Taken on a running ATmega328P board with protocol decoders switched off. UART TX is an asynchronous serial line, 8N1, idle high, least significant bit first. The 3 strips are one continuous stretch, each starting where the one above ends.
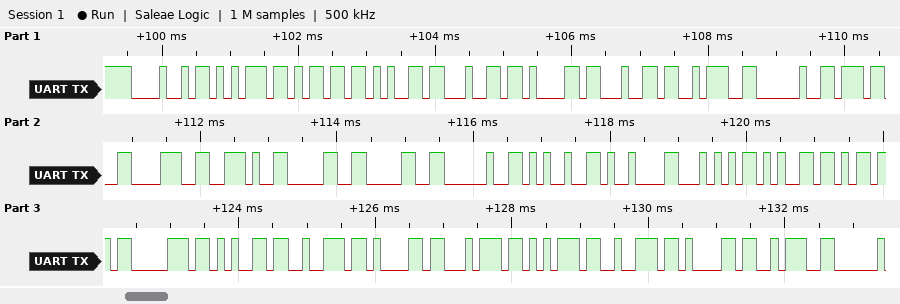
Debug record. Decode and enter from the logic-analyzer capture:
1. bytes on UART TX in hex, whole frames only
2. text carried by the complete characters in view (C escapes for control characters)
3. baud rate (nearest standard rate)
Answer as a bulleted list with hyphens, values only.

- 48 75 6D 65 64 61 64 3A 20 37 38 2E 30 30 20 25 09 54 65 6D 70 65 72 61 74 75 72 61 3A
- "Humedad: 78.00 %\tTemperatura:"
- 9600 baud
